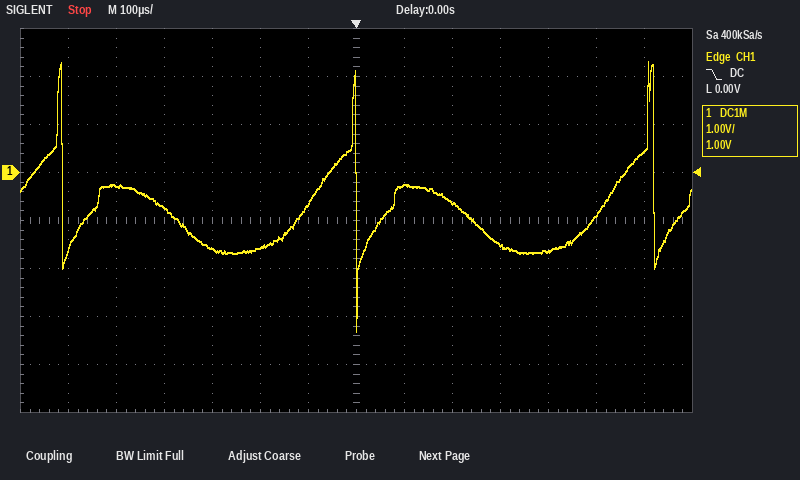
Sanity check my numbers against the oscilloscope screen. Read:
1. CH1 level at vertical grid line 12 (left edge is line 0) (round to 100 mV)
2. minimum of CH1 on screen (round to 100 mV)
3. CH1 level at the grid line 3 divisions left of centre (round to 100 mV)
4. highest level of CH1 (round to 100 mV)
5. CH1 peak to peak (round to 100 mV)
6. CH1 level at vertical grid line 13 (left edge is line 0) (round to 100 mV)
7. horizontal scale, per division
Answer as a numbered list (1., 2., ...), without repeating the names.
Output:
1. -900 mV
2. -3.3 V
3. -1.6 V
4. 2.3 V
5. 5.6 V
6. 400 mV
7. 100 µs
